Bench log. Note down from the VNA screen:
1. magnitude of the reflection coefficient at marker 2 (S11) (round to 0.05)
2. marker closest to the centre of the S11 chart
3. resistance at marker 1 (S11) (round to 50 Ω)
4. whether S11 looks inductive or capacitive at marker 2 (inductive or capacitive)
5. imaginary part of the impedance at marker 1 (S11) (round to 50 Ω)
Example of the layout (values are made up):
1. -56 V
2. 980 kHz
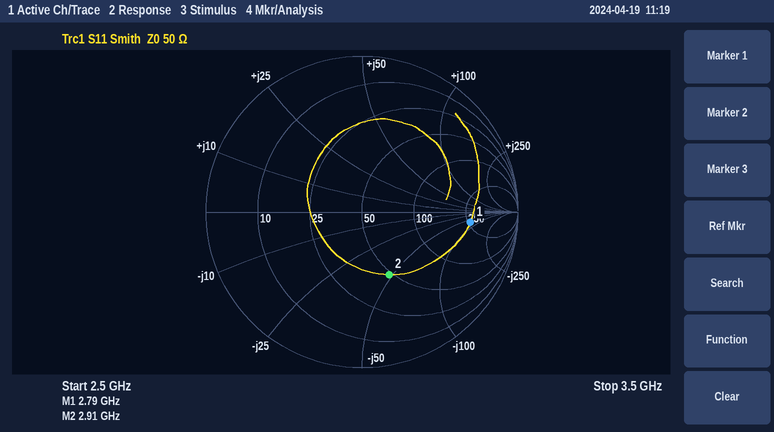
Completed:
1. 0.45
2. marker 2
3. 250 Ω
4. capacitive
5. -50 Ω
